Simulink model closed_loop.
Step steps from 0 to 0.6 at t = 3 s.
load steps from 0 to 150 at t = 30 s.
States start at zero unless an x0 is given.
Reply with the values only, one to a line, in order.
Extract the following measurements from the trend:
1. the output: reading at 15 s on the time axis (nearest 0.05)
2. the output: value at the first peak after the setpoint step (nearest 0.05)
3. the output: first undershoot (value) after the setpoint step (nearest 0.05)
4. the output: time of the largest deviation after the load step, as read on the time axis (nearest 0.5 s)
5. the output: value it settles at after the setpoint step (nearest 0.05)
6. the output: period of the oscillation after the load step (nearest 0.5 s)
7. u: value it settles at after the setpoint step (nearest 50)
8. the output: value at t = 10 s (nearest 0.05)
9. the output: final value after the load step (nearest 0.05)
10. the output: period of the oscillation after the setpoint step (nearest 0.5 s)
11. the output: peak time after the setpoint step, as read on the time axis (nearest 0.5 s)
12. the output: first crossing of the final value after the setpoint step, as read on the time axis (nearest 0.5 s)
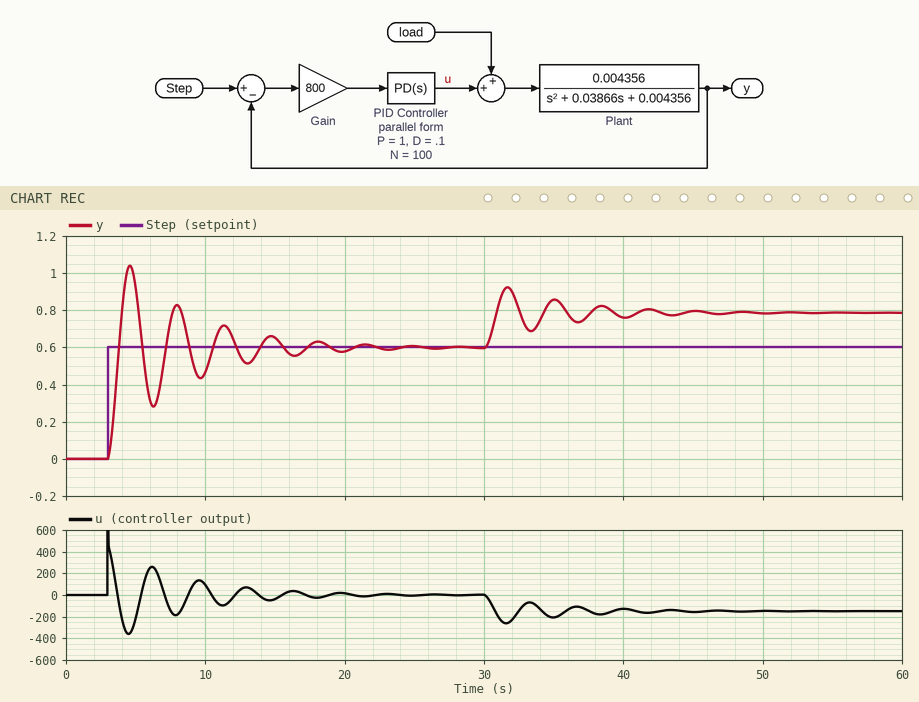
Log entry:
0.65
1.05
0.30
31.5 s
0.60
3.5 s
0
0.45
0.80
3.5 s
4.5 s
4.0 s
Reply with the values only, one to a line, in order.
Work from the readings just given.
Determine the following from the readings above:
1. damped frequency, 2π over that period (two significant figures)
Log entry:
1.8 rad/s
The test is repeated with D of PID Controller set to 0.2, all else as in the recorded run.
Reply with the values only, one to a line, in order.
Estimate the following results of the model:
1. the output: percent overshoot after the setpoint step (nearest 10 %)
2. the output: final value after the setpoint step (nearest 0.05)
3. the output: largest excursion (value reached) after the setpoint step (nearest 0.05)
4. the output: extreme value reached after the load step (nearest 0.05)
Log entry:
60 %
0.60
0.95
0.90
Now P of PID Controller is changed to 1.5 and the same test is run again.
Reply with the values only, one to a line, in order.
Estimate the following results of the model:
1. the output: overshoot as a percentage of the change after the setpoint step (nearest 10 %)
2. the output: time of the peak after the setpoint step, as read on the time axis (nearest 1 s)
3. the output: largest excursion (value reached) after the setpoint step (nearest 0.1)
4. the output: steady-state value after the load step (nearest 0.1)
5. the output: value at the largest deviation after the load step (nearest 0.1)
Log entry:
80 %
4 s
1.1
0.7
0.8
